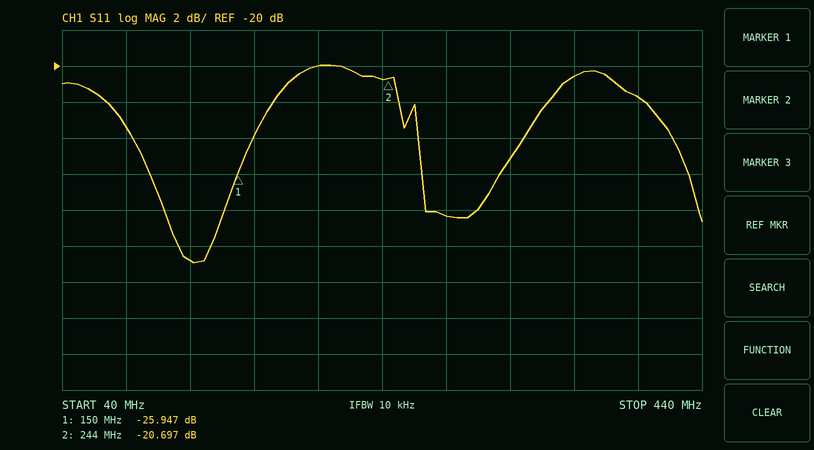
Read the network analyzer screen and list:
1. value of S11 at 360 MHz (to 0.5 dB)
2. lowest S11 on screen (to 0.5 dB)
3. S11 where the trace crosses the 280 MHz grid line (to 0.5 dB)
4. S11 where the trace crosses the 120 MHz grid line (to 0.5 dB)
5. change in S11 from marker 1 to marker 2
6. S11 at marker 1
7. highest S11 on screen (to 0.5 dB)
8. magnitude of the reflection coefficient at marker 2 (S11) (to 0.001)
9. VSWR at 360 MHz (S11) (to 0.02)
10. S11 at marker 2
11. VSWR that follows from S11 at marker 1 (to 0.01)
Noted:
-20.5 dB
-31.0 dB
-28.5 dB
-31.0 dB
5.250 dB
-25.947 dB
-20.0 dB
0.092
1.20
-20.697 dB
1.11
